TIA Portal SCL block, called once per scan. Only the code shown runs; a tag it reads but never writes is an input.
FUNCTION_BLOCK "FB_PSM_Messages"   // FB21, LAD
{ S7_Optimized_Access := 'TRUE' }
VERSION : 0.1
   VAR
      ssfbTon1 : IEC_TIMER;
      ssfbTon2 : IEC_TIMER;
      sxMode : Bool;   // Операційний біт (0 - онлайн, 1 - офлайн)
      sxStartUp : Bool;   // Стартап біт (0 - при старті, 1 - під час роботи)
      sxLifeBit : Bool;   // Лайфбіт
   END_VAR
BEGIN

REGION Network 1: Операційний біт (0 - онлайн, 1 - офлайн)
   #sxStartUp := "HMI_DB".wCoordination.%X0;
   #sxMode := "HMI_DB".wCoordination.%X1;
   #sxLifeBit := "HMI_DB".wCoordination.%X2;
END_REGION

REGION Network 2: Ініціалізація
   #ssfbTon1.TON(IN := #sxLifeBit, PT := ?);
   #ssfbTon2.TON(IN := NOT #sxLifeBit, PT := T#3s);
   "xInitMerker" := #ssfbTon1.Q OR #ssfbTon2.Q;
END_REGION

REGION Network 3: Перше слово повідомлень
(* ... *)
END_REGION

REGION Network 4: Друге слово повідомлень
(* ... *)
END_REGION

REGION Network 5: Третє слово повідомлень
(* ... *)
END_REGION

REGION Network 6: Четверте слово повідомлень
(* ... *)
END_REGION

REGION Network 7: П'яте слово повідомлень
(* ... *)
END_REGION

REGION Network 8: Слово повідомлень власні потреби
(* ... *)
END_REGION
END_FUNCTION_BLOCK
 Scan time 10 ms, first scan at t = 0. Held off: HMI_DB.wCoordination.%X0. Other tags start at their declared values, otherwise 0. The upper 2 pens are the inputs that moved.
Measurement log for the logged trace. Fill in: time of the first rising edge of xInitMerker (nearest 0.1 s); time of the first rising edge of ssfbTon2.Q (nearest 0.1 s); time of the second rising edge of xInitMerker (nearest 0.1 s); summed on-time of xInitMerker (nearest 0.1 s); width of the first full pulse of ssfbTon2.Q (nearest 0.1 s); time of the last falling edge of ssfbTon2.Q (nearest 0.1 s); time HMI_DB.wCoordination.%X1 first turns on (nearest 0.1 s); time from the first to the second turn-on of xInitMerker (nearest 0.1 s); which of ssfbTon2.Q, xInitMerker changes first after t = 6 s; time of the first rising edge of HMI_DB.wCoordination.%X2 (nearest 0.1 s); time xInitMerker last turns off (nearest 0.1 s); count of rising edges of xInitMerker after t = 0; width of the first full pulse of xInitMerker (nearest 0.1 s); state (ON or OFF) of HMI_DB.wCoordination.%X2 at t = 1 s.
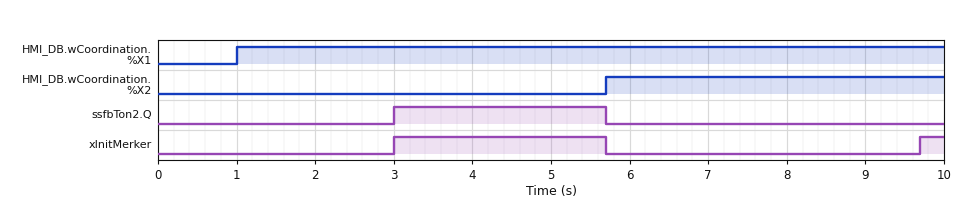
3.0 s
3.0 s
9.7 s
3.0 s
2.7 s
5.7 s
1.0 s
6.7 s
xInitMerker
5.7 s
5.7 s
2
2.7 s
OFF
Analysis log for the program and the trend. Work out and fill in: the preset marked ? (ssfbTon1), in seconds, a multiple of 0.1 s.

4.0 s
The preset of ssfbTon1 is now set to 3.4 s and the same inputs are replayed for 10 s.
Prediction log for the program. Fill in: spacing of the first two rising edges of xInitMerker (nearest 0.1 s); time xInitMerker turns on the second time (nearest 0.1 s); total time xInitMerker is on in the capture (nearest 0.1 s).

6.1 s
9.1 s
3.6 s
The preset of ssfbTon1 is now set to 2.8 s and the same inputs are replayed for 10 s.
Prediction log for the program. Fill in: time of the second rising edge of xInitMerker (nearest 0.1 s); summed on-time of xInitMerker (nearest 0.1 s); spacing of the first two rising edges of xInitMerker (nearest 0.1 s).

8.5 s
4.2 s
5.5 s
